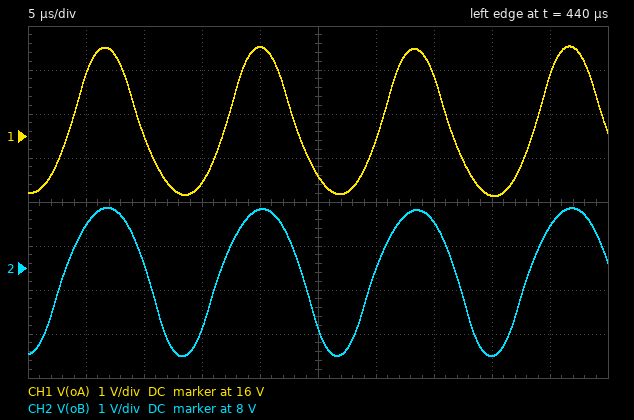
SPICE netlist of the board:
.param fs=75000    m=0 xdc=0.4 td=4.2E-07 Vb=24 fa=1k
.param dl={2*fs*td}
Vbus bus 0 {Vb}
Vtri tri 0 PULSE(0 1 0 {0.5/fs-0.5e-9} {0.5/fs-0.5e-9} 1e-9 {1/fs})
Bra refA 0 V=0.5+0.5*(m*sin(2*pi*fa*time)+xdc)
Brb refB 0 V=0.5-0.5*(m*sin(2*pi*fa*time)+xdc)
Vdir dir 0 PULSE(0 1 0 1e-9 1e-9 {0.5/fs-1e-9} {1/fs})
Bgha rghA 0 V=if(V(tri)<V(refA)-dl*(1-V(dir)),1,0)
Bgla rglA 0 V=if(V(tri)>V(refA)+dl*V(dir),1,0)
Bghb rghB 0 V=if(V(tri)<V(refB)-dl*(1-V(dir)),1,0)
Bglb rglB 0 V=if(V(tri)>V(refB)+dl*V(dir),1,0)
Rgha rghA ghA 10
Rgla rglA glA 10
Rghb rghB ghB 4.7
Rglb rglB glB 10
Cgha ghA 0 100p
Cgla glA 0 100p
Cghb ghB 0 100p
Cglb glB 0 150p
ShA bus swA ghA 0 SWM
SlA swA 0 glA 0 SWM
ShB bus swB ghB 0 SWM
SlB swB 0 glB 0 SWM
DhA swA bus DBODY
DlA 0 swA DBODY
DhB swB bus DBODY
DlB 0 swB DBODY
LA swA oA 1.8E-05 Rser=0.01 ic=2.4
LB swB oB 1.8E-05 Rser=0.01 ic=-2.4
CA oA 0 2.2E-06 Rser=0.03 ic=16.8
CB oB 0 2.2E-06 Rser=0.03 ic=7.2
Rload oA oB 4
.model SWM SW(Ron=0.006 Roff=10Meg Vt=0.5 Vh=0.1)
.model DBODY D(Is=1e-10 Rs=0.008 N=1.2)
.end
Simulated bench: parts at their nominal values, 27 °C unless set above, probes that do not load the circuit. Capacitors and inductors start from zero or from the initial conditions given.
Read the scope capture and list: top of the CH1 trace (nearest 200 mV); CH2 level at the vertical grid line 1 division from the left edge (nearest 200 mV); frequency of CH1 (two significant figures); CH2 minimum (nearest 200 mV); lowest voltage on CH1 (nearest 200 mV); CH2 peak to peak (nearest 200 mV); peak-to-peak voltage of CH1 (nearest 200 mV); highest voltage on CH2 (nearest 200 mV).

18.0 V
9.0 V
75 kHz
6.0 V
14.6 V
3.4 V
3.4 V
9.4 V
